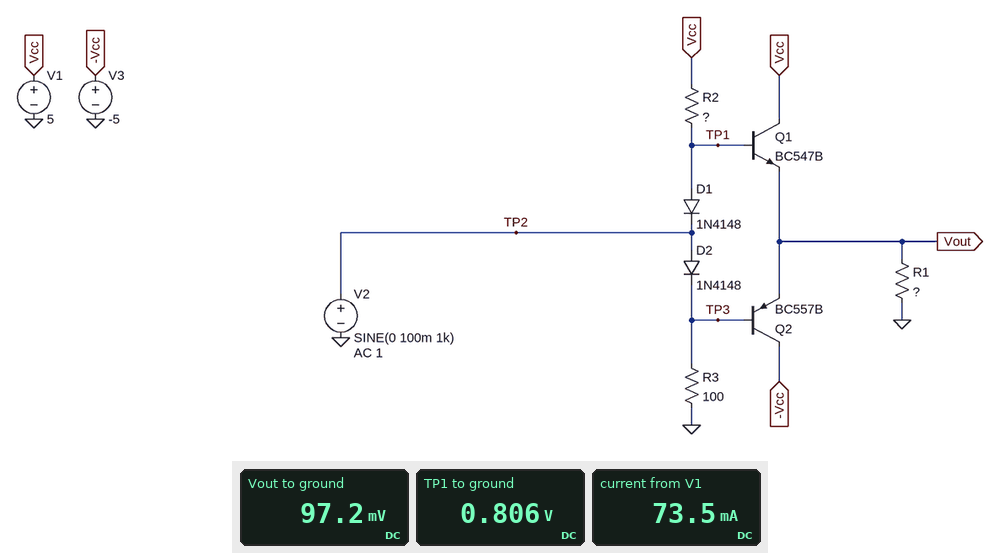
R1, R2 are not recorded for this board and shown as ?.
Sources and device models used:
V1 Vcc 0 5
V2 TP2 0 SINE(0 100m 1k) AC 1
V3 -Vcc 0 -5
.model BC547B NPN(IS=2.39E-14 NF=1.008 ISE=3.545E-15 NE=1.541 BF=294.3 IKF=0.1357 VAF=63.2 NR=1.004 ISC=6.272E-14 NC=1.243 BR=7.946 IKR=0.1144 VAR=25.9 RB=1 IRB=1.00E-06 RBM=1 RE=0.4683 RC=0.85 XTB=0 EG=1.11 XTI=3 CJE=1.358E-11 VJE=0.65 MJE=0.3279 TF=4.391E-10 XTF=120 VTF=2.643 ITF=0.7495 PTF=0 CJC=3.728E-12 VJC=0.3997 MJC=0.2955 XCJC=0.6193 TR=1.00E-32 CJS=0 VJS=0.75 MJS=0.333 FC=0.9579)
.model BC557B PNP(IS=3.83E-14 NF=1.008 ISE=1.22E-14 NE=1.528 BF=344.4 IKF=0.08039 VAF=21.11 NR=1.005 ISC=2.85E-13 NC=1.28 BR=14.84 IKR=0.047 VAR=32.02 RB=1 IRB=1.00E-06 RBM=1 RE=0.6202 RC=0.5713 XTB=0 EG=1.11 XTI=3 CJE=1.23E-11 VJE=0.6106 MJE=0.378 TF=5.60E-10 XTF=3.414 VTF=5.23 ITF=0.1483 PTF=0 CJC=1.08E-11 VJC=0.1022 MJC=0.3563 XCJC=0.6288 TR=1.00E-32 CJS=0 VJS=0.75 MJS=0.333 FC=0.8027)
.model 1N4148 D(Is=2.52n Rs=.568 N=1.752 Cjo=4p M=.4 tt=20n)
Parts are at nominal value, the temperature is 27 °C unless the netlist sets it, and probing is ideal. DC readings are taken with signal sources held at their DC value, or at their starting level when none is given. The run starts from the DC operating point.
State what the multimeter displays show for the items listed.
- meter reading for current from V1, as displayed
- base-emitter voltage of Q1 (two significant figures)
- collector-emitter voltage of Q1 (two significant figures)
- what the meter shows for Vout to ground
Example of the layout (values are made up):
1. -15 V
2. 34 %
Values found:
1. 73.5 mA
2. 710 mV
3. 4.9 V
4. 97.2 mV
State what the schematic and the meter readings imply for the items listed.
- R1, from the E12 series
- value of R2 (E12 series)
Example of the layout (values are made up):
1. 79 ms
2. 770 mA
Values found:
1. 8.2 Ω
2. 68 Ω
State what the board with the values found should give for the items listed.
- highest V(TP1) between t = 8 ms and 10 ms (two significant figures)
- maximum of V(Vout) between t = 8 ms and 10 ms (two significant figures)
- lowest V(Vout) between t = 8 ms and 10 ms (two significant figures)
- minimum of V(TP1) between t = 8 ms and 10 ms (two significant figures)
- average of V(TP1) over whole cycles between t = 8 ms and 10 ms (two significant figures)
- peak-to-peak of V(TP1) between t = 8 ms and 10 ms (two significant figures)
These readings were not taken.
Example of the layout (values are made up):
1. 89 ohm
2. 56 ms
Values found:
1. 900 mV
2. 170 mV
3. 33 mV
4. 710 mV
5. 810 mV
6. 200 mV
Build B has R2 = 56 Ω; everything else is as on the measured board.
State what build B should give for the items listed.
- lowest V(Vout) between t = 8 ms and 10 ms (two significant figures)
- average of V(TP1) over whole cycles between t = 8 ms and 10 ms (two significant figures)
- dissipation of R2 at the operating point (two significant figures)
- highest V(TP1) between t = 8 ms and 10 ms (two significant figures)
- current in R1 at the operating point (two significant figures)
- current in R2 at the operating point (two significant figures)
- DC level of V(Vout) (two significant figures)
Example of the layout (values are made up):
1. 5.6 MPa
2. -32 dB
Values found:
1. 42 mV
2. 820 mV
3. 310 mW
4. 920 mV
5. 13 mA
6. 75 mA
7. 110 mV
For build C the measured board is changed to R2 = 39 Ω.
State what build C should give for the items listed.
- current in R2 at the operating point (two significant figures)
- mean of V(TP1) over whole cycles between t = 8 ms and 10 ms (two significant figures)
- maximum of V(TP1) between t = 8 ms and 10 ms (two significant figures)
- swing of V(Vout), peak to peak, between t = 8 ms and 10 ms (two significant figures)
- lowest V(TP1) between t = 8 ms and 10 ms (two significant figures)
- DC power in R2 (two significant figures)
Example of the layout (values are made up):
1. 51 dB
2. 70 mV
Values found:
1. 110 mA
2. 860 mV
3. 950 mV
4. 150 mV
5. 760 mV
6. 440 mW
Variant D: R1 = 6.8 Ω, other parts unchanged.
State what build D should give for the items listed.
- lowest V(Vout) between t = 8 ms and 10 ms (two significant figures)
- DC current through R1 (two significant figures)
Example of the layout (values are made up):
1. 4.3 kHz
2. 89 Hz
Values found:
1. 30 mV
2. 14 mA
